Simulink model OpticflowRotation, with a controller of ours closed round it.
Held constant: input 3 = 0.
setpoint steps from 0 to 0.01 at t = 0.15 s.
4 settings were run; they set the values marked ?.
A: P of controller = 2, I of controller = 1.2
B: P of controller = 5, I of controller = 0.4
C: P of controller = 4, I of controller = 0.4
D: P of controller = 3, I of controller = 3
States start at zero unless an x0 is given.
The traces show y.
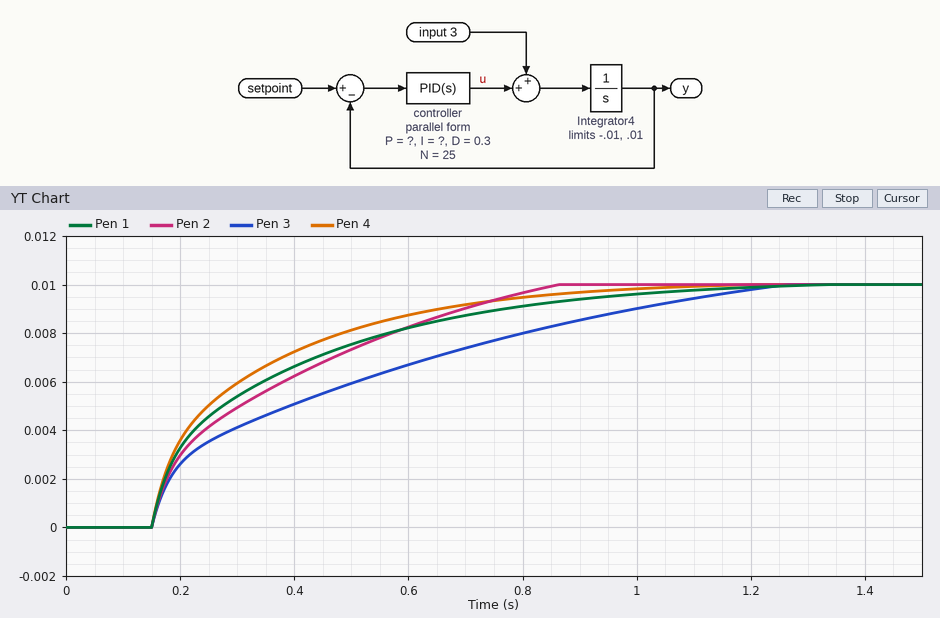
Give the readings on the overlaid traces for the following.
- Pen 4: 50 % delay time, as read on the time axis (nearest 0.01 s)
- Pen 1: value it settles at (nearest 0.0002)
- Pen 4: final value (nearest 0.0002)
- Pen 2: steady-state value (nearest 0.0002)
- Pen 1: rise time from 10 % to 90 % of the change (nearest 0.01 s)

0.25 s
0.0100
0.0100
0.0100
0.61 s
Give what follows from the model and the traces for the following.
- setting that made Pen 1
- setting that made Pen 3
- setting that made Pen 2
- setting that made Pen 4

C
A
D
B
